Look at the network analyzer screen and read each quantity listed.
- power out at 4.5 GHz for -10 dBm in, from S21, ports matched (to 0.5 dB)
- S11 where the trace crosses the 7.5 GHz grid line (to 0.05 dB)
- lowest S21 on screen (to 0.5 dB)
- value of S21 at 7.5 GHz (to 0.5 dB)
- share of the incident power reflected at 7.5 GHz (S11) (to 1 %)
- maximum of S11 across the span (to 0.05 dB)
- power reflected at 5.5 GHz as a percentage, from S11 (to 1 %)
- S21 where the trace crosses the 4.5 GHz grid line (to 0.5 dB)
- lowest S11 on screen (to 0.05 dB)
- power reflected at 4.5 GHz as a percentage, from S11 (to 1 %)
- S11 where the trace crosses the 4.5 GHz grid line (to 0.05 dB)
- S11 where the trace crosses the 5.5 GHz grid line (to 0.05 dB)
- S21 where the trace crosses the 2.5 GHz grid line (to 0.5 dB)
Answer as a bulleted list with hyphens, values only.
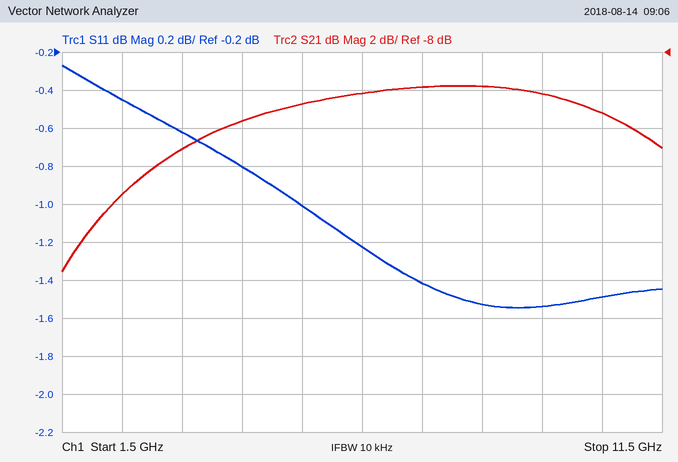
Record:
- -21.5 dBm
- -1.40 dB
- -19.5 dB
- -10.0 dB
- 72 %
- -0.25 dB
- 79 %
- -11.5 dB
- -1.55 dB
- 83 %
- -0.80 dB
- -1.00 dB
- -15.5 dB
